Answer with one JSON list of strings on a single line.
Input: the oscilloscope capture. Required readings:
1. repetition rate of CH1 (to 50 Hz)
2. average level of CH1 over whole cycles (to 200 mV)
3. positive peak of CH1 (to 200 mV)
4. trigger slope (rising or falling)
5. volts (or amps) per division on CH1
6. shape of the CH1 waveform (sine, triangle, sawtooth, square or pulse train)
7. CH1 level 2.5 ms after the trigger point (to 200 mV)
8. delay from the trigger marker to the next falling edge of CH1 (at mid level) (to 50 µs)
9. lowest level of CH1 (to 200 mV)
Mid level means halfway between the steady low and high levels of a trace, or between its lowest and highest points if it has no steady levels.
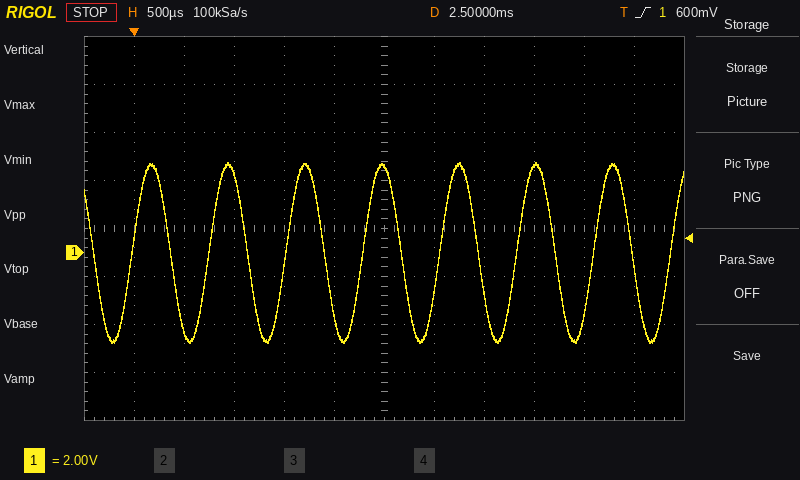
["1.30 kHz", "0.0 V", "3.8 V", "rising", "2 V", "sine", "3.6 V", "350 µs", "-3.8 V"]
